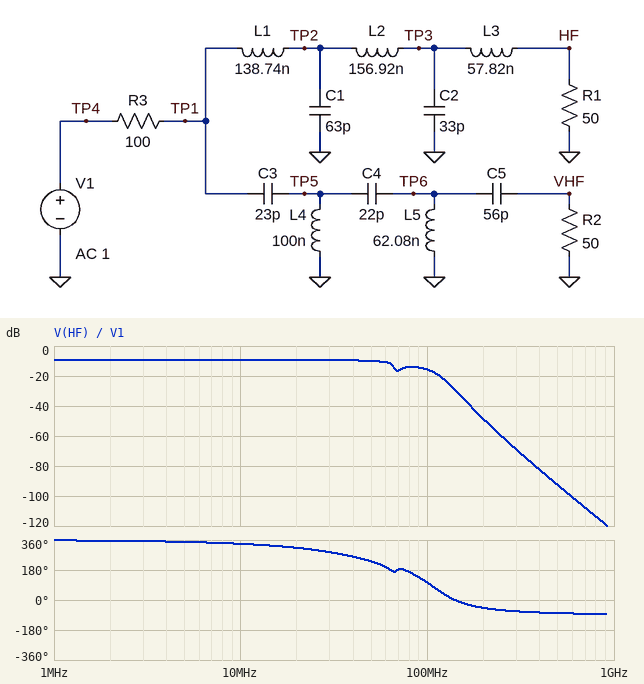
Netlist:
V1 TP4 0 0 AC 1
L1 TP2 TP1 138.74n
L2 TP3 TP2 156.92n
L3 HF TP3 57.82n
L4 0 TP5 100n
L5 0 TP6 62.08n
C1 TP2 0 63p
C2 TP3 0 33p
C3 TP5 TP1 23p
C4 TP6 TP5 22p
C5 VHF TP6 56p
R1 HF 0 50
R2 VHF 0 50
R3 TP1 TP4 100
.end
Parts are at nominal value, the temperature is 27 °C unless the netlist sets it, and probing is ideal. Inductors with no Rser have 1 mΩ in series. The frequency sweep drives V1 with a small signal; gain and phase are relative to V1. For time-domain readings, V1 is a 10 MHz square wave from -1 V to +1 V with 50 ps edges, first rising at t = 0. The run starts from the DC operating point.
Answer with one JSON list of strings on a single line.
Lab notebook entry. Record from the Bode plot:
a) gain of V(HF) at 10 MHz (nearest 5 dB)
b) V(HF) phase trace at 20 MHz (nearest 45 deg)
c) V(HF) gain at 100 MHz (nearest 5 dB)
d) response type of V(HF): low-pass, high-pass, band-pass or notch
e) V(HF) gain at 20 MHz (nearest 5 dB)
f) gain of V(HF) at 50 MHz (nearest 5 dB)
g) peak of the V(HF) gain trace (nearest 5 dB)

["-10 dB", "315 deg", "-15 dB", "low-pass", "-10 dB", "-10 dB", "-10 dB"]
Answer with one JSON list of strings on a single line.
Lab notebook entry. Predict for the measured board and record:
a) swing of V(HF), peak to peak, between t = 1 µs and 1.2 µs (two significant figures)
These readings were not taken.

["750 mV"]
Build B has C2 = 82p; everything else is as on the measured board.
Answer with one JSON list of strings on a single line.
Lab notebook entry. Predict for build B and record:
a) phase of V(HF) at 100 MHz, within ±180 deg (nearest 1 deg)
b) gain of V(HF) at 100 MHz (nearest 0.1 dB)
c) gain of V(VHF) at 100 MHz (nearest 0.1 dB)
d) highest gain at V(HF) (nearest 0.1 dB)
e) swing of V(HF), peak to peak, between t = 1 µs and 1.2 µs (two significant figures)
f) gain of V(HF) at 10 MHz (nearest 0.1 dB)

["29 deg", "-22.0 dB", "-11.7 dB", "-9.1 dB", "770 mV", "-9.6 dB"]
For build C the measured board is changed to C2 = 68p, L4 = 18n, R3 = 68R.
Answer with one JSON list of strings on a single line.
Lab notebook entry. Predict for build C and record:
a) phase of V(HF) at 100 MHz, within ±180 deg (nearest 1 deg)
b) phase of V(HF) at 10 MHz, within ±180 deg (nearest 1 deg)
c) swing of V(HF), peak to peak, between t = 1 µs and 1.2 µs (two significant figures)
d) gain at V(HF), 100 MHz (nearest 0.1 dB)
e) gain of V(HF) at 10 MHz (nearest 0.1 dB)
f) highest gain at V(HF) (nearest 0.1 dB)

["9 deg", "-27 deg", "1.1 V", "-13.5 dB", "-7.5 dB", "-7.4 dB"]
